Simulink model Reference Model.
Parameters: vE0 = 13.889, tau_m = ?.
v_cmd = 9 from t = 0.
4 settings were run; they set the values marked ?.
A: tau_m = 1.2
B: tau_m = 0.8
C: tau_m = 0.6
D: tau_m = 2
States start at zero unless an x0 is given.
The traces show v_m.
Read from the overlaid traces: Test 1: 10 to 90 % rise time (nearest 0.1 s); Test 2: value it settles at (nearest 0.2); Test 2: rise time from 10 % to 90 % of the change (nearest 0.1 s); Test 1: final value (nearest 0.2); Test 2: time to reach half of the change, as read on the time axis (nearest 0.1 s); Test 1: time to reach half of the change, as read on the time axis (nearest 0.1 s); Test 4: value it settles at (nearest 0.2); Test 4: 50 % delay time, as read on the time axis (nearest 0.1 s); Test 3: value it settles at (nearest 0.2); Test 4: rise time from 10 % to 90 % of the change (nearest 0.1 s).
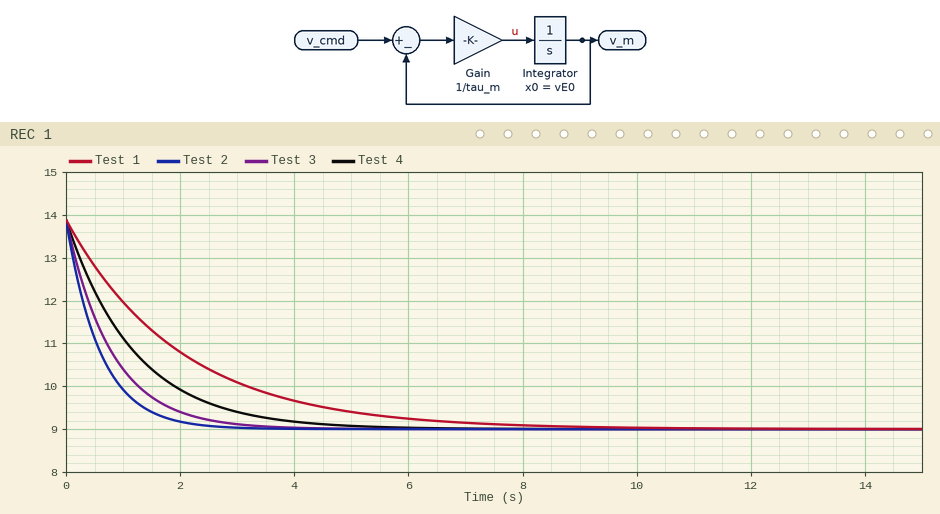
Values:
4.4 s
9.0
1.3 s
9.0
0.4 s
1.4 s
9.0
0.8 s
9.0
2.6 s
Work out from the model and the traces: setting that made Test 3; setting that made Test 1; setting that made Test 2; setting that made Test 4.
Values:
B
D
C
A
